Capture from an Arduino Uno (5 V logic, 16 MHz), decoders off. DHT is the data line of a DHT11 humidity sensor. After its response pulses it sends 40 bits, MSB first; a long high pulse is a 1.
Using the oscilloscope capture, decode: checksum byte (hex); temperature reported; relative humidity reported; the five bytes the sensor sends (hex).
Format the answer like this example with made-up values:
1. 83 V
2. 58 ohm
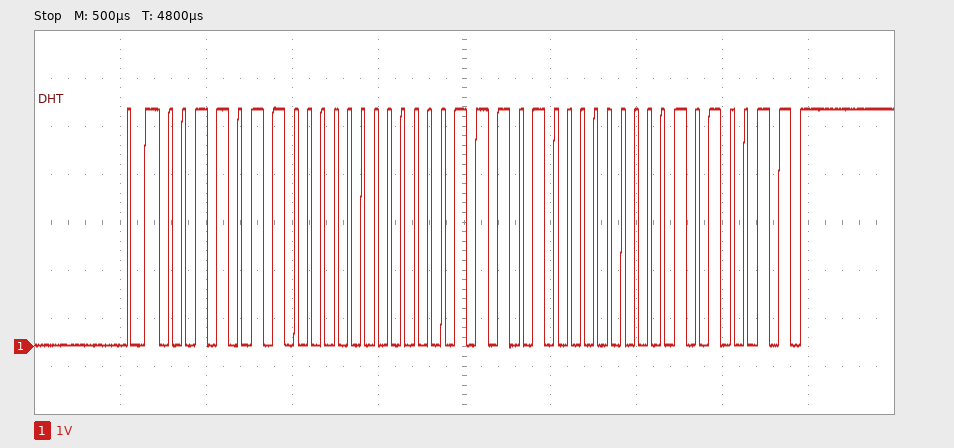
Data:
1. 0x53
2. 29.0 °C
3. 54 %
4. 36 00 1D 00 53
